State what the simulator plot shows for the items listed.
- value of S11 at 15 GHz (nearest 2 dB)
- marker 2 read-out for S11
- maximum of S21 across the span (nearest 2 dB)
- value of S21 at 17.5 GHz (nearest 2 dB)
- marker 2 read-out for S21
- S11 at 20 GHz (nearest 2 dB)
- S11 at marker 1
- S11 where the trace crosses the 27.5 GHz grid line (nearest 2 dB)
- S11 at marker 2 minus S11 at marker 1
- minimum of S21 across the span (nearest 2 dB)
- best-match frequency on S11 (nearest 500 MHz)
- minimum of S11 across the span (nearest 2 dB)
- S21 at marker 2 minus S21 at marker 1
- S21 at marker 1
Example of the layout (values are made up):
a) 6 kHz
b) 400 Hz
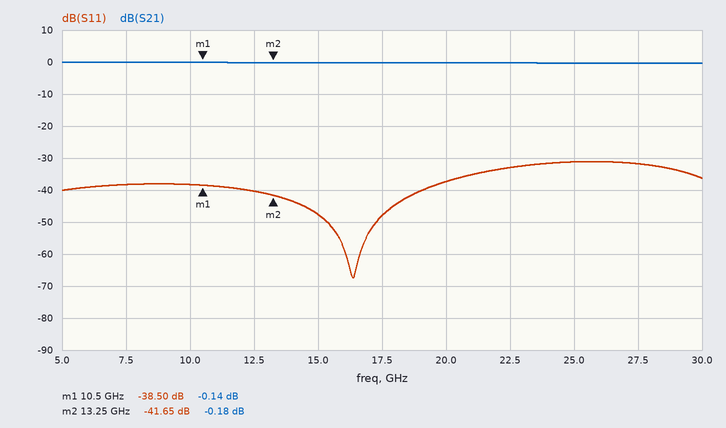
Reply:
a) -48 dB
b) -41.65 dB
c) 0 dB
d) 0 dB
e) -0.18 dB
f) -38 dB
g) -38.50 dB
h) -32 dB
i) -3.15 dB
j) 0 dB
k) 16.5 GHz
l) -68 dB
m) -0.04 dB
n) -0.14 dB
